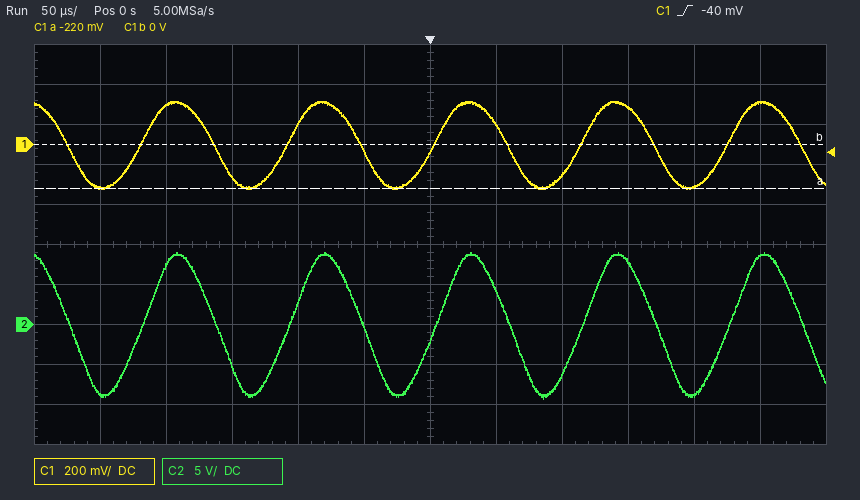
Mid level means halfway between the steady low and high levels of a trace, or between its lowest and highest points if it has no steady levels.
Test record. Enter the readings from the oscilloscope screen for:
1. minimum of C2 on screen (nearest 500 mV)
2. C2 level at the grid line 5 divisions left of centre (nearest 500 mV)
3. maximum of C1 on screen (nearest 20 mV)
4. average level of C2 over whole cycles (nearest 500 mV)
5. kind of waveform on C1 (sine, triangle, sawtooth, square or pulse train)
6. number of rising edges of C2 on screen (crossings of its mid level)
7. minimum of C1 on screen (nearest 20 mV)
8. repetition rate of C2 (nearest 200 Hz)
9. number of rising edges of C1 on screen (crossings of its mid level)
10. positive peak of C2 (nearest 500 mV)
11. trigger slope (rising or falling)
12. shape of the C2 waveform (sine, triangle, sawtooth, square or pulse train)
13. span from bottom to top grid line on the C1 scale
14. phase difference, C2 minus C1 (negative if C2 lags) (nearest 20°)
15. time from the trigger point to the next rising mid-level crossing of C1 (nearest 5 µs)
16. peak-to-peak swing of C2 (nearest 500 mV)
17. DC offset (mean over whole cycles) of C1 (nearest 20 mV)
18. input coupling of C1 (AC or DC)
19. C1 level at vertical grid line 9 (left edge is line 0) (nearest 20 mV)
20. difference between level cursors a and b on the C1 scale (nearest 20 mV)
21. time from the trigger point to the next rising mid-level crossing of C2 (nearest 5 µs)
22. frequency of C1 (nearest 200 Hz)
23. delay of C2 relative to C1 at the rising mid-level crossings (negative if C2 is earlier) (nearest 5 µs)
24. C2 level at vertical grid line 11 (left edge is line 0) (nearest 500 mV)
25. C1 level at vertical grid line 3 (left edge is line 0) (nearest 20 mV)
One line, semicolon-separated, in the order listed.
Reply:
-9.0 V; -8.5 V; 220 mV; 0.0 V; sine; 5; -220 mV; 9.0 kHz; 5; 9.0 V; rising; sine; 2 V; 0°; 5 µs; 18.0 V; 0 mV; DC; 180 mV; 220 mV; 5 µs; 9.0 kHz; 0 µs; 8.5 V; -160 mV
